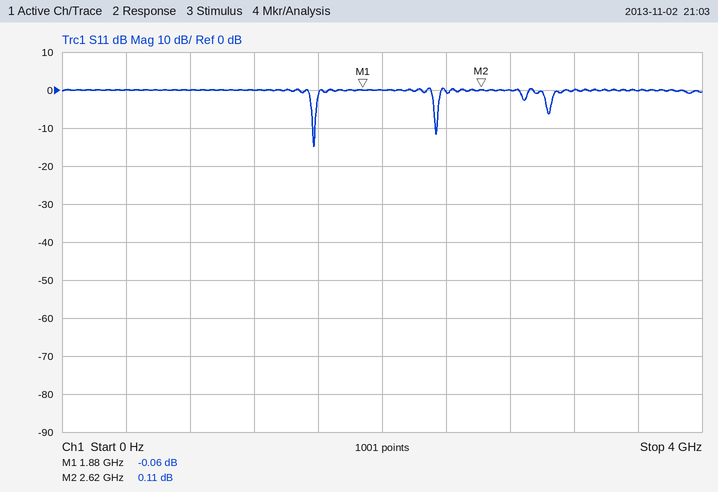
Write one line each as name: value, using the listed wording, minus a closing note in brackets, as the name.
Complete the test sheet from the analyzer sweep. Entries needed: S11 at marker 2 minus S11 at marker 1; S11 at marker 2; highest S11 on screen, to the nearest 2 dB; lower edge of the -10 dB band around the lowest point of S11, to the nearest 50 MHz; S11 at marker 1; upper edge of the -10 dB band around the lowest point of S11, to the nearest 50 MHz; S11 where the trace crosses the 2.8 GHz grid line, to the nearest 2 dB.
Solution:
S11 at marker 2 minus S11 at marker 1: 0.17 dB
S11 at marker 2: 0.11 dB
highest S11 on screen, to the nearest 2 dB: 0 dB
lower edge of the -10 dB band around the lowest point of S11, to the nearest 50 MHz: 1.55 GHz
S11 at marker 1: -0.06 dB
upper edge of the -10 dB band around the lowest point of S11, to the nearest 50 MHz: 1.60 GHz
S11 where the trace crosses the 2.8 GHz grid line, to the nearest 2 dB: 0 dB
